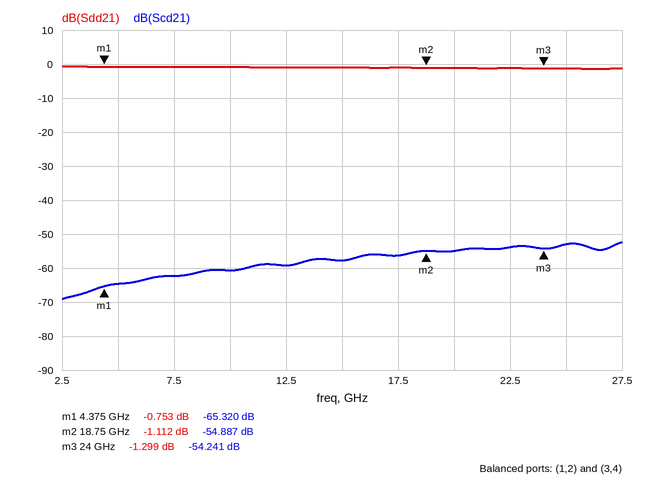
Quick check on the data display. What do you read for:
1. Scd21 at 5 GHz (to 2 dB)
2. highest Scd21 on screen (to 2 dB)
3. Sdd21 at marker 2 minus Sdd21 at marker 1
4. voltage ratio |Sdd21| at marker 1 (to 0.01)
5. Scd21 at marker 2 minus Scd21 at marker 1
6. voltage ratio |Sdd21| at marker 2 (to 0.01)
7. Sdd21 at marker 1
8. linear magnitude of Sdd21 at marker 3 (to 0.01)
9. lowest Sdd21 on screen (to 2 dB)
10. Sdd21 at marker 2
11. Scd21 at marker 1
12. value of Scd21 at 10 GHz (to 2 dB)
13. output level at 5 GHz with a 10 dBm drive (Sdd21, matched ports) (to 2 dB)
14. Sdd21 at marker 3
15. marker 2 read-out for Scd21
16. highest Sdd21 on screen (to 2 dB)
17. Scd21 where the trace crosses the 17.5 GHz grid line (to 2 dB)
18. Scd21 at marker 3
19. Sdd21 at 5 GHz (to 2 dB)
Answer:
-64 dB
-52 dB
-0.359 dB
0.92
10.433 dB
0.88
-0.753 dB
0.86
-2 dB
-1.112 dB
-65.320 dB
-60 dB
10 dBm
-1.299 dB
-54.887 dB
0 dB
-56 dB
-54.241 dB
0 dB
